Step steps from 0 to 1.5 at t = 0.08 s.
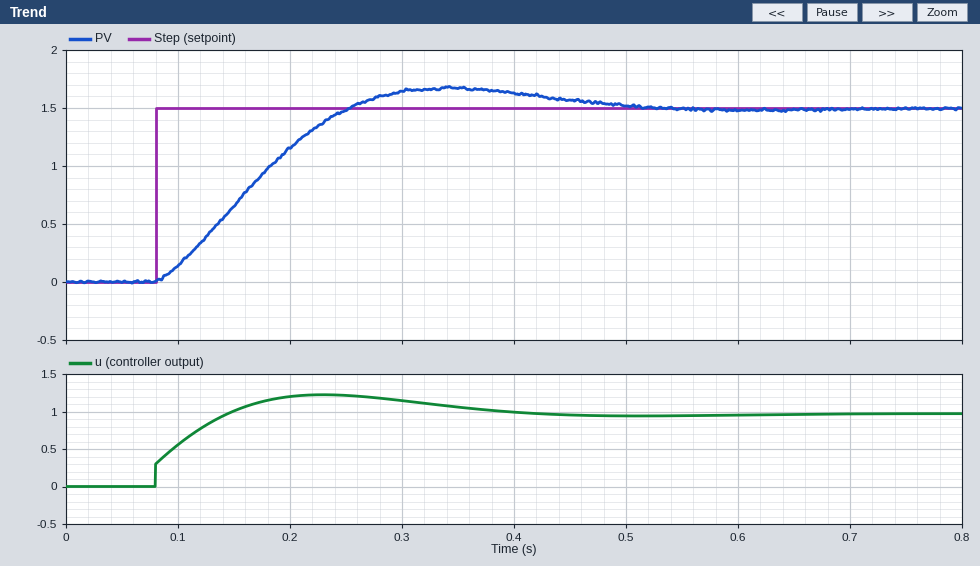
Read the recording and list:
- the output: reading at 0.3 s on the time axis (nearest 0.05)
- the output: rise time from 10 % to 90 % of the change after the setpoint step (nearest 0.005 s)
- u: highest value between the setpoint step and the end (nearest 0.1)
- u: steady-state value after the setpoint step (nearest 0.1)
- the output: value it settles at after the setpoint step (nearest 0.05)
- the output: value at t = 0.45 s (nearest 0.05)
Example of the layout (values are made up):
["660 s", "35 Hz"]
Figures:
["1.65", "0.125 s", "1.2", "1.0", "1.50", "1.55"]
